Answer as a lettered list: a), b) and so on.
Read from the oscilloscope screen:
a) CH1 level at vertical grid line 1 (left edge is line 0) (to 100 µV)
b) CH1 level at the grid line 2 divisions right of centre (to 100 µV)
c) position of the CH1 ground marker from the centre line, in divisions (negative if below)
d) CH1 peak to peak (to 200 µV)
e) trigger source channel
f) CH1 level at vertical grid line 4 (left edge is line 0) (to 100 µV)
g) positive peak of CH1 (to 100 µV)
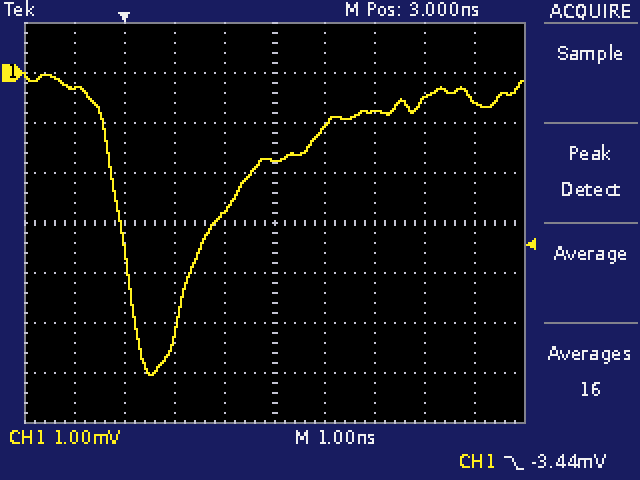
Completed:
a) -300 µV
b) -800 µV
c) +3.0 div
d) 6.0 mV
e) CH1
f) -2.8 mV
g) 0.0 mV
